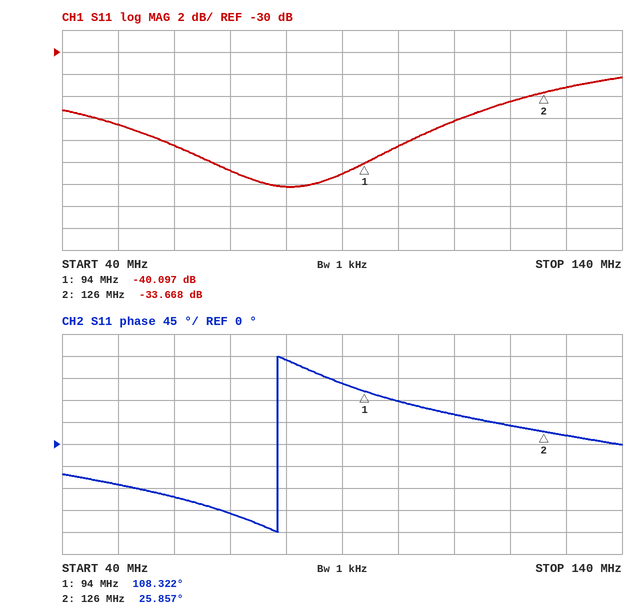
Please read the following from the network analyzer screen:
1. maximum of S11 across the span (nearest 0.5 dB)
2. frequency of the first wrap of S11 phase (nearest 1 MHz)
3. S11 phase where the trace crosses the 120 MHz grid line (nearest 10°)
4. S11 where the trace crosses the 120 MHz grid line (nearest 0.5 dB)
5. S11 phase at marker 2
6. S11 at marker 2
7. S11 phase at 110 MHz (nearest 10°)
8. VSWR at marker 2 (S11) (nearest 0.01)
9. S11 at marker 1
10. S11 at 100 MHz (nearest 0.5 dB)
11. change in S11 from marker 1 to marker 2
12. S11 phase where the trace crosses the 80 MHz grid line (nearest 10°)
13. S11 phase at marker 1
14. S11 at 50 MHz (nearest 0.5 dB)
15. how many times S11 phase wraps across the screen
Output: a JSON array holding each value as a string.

["-32.5 dB", "79 MHz", "40°", "-34.5 dB", "25.857°", "-33.668 dB", "60°", "1.04", "-40.097 dB", "-38.5 dB", "6.429 dB", "170°", "108.322°", "-36.5 dB", "1"]
